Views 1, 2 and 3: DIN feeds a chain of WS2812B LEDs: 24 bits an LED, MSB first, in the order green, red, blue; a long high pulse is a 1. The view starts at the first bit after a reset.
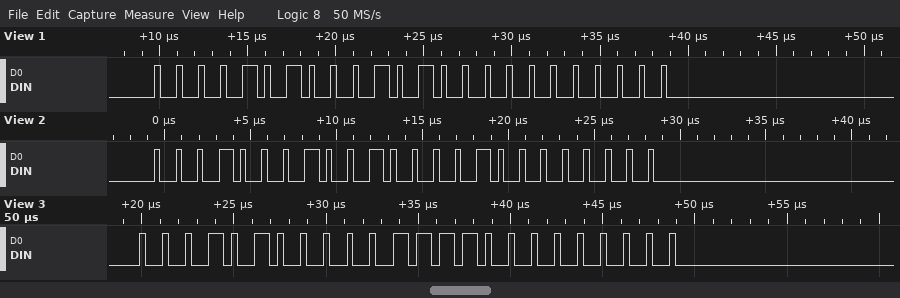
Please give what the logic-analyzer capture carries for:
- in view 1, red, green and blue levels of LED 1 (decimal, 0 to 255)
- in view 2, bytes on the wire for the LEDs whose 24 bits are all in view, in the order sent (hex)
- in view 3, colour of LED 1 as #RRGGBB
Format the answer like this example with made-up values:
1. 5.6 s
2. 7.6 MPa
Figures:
1. 40, 10, 0
2. 11 21 00
3. #1E1400
